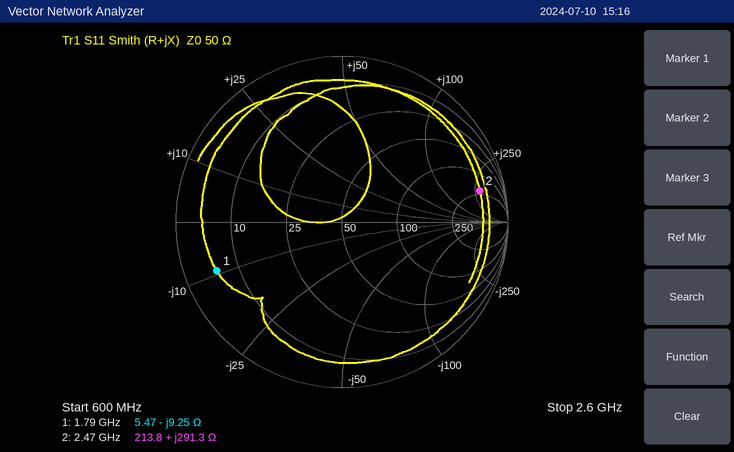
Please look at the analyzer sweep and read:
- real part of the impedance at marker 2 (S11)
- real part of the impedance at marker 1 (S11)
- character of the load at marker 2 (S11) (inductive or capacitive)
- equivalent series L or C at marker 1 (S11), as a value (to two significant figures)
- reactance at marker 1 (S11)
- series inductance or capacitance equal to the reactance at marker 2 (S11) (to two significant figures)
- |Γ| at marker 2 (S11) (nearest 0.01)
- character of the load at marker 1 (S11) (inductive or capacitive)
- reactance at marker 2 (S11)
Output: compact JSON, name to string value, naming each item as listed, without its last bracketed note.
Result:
{"real part of the impedance at marker 2": "213.8 Ω", "real part of the impedance at marker 1": "5.47 Ω", "character of the load at marker 2 (S11)": "inductive", "equivalent series L or C at marker 1 (S11), as a value": "9.6 pF", "reactance at marker 1": "-9.25 Ω", "series inductance or capacitance equal to the reactance at marker 2 (S11)": "19 nH", "|Γ| at marker 2 (S11)": "0.85", "character of the load at marker 1 (S11)": "capacitive", "reactance at marker 2": "+291.3 Ω"}
